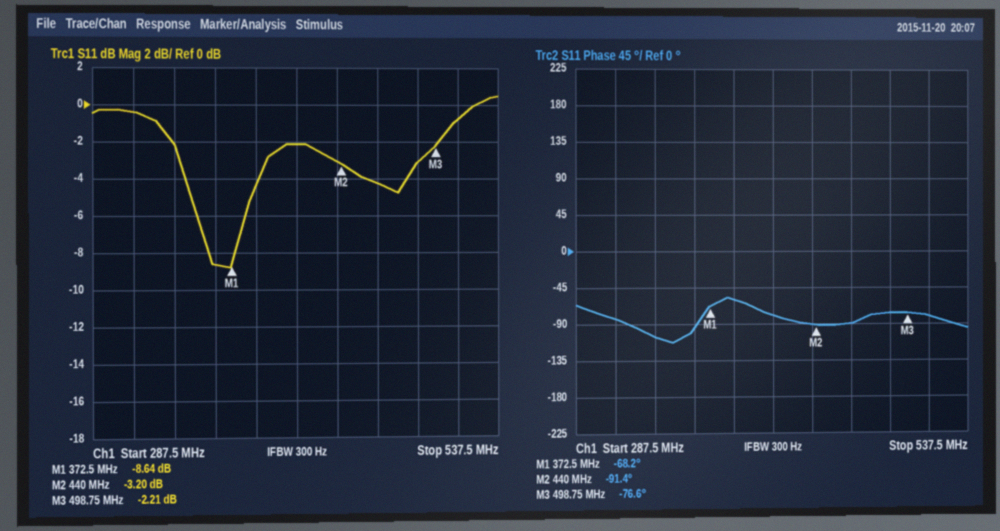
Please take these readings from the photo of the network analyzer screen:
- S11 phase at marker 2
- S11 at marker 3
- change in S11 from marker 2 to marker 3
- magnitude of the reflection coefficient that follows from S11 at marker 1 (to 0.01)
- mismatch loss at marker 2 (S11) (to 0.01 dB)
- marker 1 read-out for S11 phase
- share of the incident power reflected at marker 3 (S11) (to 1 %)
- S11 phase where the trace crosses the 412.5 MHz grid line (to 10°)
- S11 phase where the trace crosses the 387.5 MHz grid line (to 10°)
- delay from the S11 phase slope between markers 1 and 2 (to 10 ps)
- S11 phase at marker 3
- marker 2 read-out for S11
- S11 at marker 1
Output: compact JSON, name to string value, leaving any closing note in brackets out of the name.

{"S11 phase at marker 2": "-91.4°", "S11 at marker 3": "-2.21 dB", "change in S11 from marker 2 to marker 3": "0.99 dB", "magnitude of the reflection coefficient that follows from S11 at marker 1": "0.37", "mismatch loss at marker 2 (S11)": "2.83 dB", "marker 1 read-out for S11 phase": "-68.2°", "share of the incident power reflected at marker 3 (S11)": "60 %", "S11 phase where the trace crosses the 412.5 MHz grid line": "-80°", "S11 phase where the trace crosses the 387.5 MHz grid line": "-60°", "delay from the S11 phase slope between markers 1 and 2": "950 ps", "S11 phase at marker 3": "-76.6°", "marker 2 read-out for S11": "-3.20 dB", "S11 at marker 1": "-8.64 dB"}
